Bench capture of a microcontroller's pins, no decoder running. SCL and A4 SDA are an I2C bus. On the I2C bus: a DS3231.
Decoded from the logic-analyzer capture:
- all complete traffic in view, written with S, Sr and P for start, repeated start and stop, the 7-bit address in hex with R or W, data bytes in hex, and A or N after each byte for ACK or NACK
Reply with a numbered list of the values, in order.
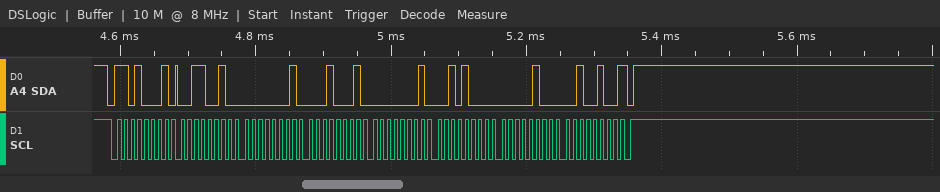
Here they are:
1. S 68R A 32 A 01 A 11 A 01 A 28 A 04 A 24 N P
